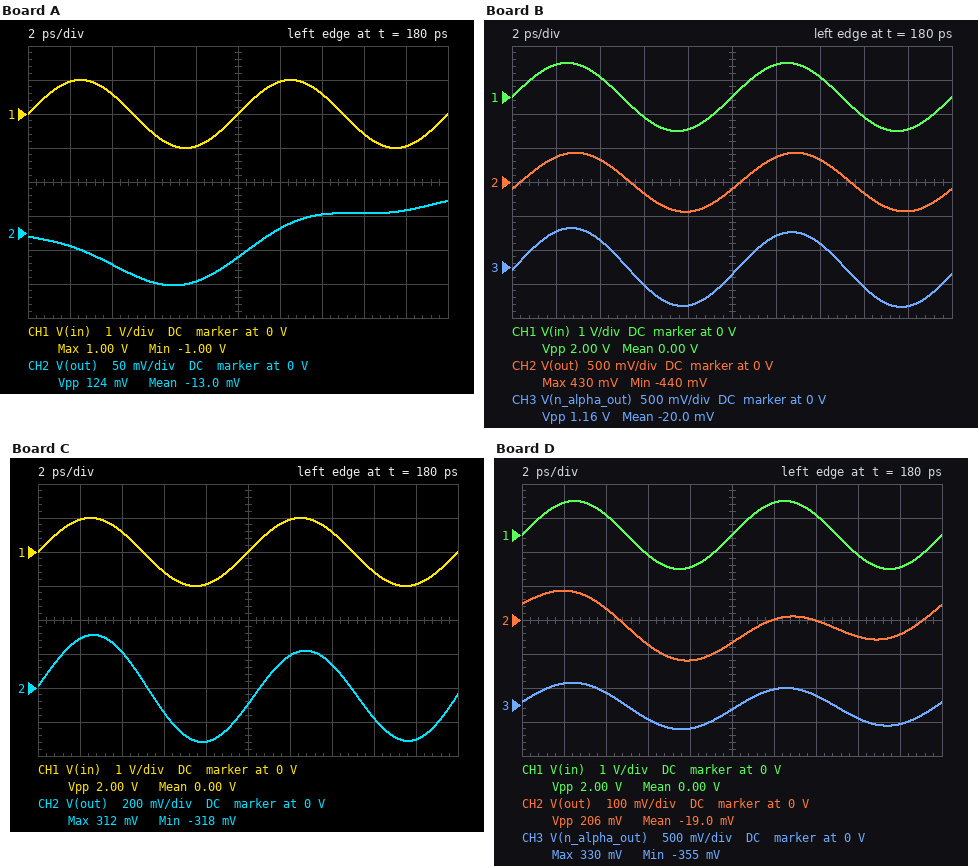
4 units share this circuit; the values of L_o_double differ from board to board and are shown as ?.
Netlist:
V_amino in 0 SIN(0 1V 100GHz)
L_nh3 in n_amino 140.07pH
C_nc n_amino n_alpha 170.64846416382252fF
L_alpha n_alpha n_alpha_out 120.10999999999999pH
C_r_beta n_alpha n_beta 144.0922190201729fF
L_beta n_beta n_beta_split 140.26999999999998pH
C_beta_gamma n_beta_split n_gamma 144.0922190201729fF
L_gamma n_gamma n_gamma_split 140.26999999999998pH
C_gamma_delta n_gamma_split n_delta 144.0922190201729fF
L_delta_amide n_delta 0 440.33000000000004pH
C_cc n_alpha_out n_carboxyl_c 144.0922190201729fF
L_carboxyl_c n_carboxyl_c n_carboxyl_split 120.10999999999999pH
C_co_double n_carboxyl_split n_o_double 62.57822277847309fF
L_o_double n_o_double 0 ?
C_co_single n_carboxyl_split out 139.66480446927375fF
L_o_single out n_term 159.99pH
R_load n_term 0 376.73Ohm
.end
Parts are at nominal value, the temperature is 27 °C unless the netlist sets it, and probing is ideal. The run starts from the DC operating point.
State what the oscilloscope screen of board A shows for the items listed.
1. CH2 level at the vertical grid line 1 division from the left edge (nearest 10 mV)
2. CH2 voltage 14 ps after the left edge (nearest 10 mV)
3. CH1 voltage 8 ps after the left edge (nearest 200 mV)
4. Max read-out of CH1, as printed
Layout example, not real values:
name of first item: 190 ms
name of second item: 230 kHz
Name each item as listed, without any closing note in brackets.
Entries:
CH2 level at the vertical grid line 1 division from the left edge: -20 mV
CH2 voltage 14 ps after the left edge: 30 mV
CH1 voltage 8 ps after the left edge: -1.0 V
Max read-out of CH1, as printed: 1.00 V
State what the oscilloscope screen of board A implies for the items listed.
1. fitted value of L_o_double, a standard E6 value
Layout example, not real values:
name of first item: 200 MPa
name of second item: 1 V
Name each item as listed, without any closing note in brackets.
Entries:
fitted value of L_o_double, a standard E6 value: 47 pH
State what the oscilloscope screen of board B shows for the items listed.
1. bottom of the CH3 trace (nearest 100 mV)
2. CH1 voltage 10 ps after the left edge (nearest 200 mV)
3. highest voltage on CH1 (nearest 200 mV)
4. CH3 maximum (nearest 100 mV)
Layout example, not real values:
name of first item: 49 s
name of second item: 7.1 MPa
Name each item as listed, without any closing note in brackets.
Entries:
bottom of the CH3 trace: -600 mV
CH1 voltage 10 ps after the left edge: 0 V
highest voltage on CH1: 1.0 V
CH3 maximum: 600 mV
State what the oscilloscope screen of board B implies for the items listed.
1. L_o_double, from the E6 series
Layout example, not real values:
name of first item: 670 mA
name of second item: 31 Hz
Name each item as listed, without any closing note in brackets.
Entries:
L_o_double, from the E6 series: 470 pH
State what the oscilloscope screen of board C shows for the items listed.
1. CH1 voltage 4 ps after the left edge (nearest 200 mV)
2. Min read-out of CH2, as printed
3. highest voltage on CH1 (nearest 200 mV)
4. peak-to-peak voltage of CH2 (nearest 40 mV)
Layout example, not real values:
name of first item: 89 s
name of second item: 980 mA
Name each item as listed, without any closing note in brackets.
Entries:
CH1 voltage 4 ps after the left edge: 600 mV
Min read-out of CH2, as printed: -318 mV
highest voltage on CH1: 1.0 V
peak-to-peak voltage of CH2: 640 mV
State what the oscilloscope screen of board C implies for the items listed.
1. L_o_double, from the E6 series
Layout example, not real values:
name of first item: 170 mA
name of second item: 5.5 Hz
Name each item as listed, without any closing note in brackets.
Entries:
L_o_double, from the E6 series: 220 pH
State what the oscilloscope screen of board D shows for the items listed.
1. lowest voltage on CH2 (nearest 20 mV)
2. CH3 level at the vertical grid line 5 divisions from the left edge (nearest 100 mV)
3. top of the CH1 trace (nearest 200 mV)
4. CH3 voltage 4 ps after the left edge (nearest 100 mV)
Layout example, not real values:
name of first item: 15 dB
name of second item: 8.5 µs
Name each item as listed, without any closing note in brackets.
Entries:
lowest voltage on CH2: -120 mV
CH3 level at the vertical grid line 5 divisions from the left edge: -100 mV
top of the CH1 trace: 1.0 V
CH3 voltage 4 ps after the left edge: 200 mV
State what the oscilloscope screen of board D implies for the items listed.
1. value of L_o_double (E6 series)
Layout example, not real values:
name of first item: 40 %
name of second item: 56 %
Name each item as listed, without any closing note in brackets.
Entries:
value of L_o_double: 68 pH
